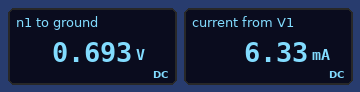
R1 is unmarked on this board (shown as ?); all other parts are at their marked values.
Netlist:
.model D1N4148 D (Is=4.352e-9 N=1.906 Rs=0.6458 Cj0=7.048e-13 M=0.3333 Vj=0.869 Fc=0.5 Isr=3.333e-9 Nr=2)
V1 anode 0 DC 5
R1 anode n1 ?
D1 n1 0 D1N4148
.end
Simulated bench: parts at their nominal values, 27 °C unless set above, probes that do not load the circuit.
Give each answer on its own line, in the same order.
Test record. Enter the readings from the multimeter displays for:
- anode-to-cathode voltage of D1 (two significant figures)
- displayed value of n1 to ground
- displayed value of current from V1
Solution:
690 mV
0.693 V
6.33 mA
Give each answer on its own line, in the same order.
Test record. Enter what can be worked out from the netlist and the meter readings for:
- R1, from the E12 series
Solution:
680 Ω
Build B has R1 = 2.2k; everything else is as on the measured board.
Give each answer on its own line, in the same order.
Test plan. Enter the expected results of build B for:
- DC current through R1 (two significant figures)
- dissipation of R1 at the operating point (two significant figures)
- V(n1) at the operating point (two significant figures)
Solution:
2.0 mA
8.7 mW
630 mV
